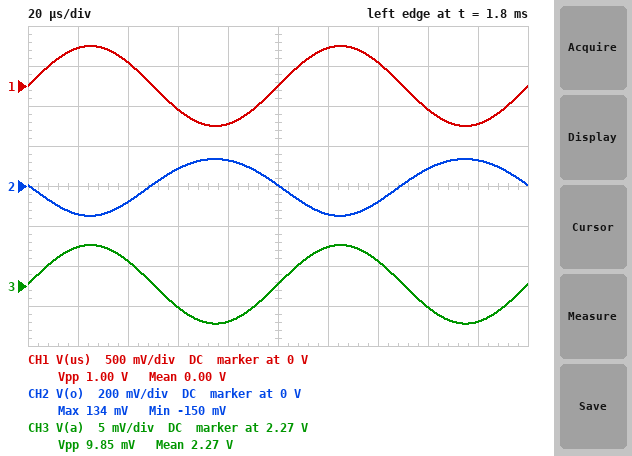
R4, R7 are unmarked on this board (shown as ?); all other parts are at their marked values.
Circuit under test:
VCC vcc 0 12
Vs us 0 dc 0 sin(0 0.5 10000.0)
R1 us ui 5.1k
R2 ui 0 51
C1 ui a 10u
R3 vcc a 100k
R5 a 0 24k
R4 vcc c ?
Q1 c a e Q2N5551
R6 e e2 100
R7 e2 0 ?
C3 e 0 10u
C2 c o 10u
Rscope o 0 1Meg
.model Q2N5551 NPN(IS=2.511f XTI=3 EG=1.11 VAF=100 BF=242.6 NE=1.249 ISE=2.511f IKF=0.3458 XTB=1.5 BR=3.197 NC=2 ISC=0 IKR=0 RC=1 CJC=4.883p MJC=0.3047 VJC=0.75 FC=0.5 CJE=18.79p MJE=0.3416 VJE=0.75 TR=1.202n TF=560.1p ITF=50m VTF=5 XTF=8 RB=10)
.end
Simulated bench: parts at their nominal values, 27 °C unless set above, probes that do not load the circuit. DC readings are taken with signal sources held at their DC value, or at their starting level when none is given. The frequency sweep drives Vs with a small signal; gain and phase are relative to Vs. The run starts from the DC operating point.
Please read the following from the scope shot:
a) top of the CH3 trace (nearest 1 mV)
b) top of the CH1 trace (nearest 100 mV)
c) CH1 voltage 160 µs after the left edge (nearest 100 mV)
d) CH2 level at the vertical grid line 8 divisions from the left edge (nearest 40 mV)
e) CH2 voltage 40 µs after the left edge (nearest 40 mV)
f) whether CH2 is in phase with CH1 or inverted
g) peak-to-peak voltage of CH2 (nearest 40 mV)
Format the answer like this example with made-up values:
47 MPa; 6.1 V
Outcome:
2.275 V; 500 mV; -300 mV; 80 mV; -80 mV; inverted; 280 mV
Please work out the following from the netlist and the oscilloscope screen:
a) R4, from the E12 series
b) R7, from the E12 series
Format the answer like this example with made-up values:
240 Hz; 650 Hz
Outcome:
2.7 kΩ; 5.6 kΩ
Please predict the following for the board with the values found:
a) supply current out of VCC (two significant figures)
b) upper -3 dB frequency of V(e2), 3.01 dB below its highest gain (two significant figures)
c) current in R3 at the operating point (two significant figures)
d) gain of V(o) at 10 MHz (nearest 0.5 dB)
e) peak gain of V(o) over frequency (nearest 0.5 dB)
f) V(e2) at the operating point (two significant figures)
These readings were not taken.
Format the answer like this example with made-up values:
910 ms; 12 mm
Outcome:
380 µA; 180 Hz; 97 µA; -12.5 dB; -11.0 dB; 1.6 V
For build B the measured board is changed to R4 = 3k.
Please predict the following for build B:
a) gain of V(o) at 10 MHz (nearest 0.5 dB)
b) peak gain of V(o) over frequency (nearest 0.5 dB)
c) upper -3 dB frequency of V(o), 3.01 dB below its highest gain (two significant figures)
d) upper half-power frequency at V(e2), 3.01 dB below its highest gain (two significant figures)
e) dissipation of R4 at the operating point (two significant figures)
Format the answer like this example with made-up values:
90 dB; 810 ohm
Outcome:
-12.0 dB; -10.0 dB; 13 MHz; 180 Hz; 240 µW
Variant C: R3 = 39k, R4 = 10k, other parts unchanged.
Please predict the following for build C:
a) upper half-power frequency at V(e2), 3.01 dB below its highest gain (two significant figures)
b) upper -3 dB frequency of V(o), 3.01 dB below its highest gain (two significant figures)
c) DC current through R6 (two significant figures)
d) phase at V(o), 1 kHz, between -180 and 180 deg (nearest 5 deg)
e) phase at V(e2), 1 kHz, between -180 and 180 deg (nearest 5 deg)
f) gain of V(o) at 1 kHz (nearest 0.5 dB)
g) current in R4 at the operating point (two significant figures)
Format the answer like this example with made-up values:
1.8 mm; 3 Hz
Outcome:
390 Hz; 1.7 MHz; 670 µA; -160 deg; -70 deg; 6.5 dB; 660 µA
